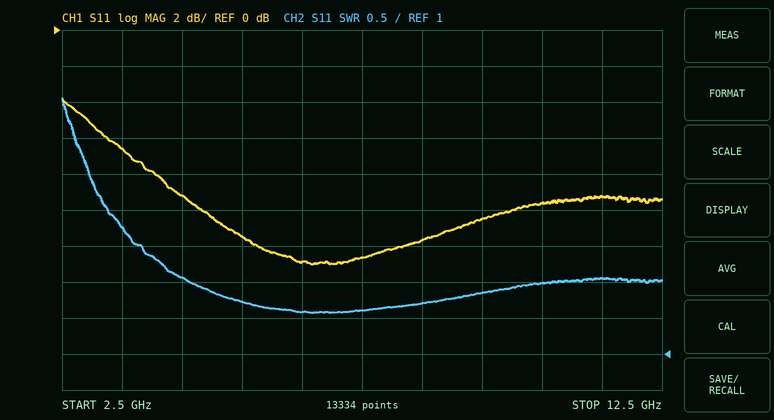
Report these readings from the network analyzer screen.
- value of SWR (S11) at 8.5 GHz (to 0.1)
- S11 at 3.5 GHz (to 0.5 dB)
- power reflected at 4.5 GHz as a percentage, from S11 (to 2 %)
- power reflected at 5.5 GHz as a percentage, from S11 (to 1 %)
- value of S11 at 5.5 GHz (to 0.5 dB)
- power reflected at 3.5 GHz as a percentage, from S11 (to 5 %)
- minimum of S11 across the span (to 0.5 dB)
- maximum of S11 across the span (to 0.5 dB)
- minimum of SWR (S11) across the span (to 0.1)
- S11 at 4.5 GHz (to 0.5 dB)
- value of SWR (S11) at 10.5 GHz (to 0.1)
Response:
1.7
-6.5 dB
12 %
7 %
-11.5 dB
20 %
-13.0 dB
-4.0 dB
1.6
-9.0 dB
2.0
